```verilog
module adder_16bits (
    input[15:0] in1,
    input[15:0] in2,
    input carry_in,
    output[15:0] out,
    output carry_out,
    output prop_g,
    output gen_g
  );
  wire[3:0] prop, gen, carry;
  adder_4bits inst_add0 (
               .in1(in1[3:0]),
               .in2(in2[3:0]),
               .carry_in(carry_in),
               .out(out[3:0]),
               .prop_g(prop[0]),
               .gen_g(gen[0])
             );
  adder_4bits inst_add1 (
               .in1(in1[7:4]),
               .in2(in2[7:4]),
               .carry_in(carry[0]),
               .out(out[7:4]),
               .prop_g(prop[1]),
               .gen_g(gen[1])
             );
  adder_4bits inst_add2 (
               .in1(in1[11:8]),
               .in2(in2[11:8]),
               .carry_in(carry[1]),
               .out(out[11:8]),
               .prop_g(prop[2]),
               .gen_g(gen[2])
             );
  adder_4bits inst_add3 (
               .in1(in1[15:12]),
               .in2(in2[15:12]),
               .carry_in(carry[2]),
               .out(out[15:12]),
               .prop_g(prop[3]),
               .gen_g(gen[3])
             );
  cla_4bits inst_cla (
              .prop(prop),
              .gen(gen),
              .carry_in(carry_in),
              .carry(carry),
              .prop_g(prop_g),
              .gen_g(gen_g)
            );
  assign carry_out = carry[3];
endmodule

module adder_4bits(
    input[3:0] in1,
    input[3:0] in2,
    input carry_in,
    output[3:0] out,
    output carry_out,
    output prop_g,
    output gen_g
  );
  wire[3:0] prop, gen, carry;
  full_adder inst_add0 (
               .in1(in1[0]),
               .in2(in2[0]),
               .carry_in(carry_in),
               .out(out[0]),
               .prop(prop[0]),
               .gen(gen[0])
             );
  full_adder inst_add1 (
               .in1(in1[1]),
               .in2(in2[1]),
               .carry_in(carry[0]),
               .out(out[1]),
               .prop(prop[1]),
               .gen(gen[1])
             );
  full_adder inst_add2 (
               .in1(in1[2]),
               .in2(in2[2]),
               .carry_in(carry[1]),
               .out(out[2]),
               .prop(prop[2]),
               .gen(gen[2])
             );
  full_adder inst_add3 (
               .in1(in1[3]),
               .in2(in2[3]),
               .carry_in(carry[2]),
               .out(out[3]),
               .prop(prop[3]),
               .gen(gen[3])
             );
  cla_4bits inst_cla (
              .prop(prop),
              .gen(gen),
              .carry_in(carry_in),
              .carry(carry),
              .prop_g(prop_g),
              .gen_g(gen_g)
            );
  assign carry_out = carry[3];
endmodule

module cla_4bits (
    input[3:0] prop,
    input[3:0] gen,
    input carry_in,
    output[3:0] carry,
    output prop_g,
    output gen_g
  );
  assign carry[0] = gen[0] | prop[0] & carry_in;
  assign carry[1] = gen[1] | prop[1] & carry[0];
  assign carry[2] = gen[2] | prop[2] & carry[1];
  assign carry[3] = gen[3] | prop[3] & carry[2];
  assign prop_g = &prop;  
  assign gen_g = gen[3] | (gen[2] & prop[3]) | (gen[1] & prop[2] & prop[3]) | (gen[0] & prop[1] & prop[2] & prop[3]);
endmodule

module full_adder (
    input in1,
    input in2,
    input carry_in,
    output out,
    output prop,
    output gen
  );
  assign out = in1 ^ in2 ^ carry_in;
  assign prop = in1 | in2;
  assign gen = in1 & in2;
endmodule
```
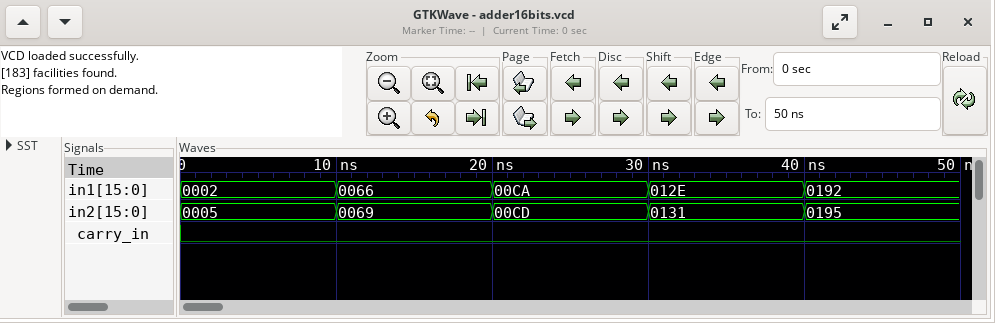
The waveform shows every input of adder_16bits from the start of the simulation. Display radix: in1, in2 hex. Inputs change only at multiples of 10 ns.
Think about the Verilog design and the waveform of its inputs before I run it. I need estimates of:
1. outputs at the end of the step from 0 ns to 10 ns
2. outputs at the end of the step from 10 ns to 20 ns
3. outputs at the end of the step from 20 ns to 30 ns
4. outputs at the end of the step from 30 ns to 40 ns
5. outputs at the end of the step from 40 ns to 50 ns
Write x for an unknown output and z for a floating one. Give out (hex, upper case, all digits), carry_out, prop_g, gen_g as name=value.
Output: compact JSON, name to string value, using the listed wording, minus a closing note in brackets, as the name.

{"outputs at the end of the step from 0 ns to 10 ns": "out=0007, carry_out=0, prop_g=0, gen_g=0", "outputs at the end of the step from 10 ns to 20 ns": "out=00CF, carry_out=0, prop_g=0, gen_g=0", "outputs at the end of the step from 20 ns to 30 ns": "out=0197, carry_out=0, prop_g=0, gen_g=0", "outputs at the end of the step from 30 ns to 40 ns": "out=025F, carry_out=0, prop_g=0, gen_g=0", "outputs at the end of the step from 40 ns to 50 ns": "out=0327, carry_out=0, prop_g=0, gen_g=0"}
